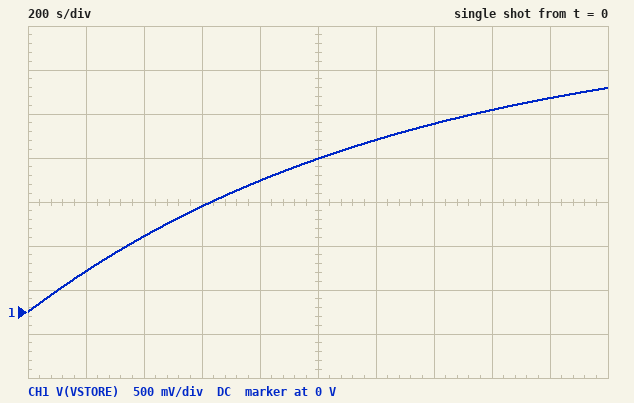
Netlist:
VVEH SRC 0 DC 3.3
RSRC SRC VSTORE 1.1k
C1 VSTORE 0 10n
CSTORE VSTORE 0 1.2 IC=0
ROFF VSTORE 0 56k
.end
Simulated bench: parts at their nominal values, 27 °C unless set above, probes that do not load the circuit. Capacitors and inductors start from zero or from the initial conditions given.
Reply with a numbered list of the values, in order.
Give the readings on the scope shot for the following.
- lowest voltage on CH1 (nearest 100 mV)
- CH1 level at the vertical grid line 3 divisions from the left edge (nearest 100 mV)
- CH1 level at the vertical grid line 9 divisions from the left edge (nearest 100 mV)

1. 0 V
2. 1.2 V
3. 2.4 V
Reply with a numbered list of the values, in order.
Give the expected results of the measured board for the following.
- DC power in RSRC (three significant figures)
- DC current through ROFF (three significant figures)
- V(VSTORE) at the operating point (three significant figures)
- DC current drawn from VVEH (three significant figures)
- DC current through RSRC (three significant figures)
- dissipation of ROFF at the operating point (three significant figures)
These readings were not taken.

1. 3.67 µW
2. 57.8 µA
3. 3.24 V
4. 57.8 µA
5. 57.8 µA
6. 187 µW
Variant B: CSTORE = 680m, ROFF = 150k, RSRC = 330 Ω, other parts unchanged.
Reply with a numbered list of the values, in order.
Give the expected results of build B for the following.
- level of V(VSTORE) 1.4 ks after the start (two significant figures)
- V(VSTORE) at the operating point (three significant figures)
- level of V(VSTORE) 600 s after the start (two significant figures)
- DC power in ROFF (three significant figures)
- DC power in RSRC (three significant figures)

1. 3.3 V
2. 3.29 V
3. 3.1 V
4. 72.3 µW
5. 159 nW
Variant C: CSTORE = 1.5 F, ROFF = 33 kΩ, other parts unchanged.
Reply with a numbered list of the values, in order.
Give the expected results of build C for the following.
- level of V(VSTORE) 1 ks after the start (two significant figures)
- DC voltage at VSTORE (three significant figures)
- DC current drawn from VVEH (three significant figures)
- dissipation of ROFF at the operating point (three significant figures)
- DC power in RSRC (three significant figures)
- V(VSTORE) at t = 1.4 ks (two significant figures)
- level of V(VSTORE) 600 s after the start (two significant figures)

1. 1.5 V
2. 3.19 V
3. 96.8 µA
4. 309 µW
5. 10.3 µW
6. 1.9 V
7. 1.0 V
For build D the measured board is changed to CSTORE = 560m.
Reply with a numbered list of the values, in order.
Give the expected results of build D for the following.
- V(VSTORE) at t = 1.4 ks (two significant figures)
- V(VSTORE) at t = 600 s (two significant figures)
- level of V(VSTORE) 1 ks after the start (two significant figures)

1. 2.9 V
2. 2.0 V
3. 2.6 V
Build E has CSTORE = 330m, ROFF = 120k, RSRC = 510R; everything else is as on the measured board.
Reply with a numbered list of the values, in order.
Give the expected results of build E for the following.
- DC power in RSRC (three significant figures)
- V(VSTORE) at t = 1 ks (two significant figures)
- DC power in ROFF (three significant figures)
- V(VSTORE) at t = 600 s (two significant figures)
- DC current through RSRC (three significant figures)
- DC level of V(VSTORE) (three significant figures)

1. 382 nW
2. 3.3 V
3. 90.0 µW
4. 3.2 V
5. 27.4 µA
6. 3.29 V
